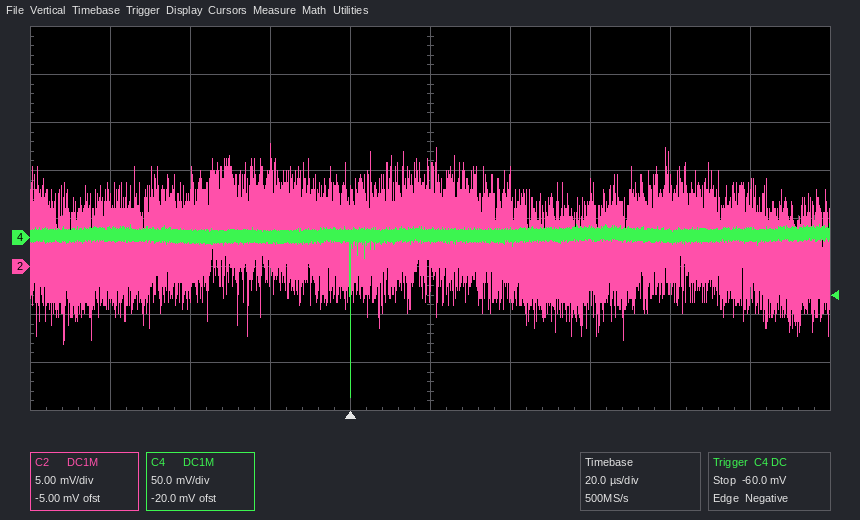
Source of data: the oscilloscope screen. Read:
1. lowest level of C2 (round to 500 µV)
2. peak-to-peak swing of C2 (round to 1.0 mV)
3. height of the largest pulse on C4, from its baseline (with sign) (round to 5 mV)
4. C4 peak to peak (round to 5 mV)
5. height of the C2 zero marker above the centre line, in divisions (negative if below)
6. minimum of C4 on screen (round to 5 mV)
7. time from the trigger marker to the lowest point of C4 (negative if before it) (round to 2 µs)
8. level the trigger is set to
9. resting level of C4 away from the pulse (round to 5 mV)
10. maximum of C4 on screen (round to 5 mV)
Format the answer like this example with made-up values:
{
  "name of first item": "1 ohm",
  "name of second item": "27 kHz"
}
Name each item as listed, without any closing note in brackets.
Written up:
{
  "lowest level of C2": "-8.0 mV",
  "peak-to-peak swing of C2": "21.0 mV",
  "height of the largest pulse on C4, from its baseline (with sign)": "-170 mV",
  "C4 peak to peak": "180 mV",
  "height of the C2 zero marker above the centre line, in divisions": "-1.0 div",
  "minimum of C4 on screen": "-165 mV",
  "time from the trigger marker to the lowest point of C4 (negative if before it)": "0 µs",
  "level the trigger is set to": "-60.0 mV",
  "resting level of C4 away from the pulse": "5 mV",
  "maximum of C4 on screen": "15 mV"
}
